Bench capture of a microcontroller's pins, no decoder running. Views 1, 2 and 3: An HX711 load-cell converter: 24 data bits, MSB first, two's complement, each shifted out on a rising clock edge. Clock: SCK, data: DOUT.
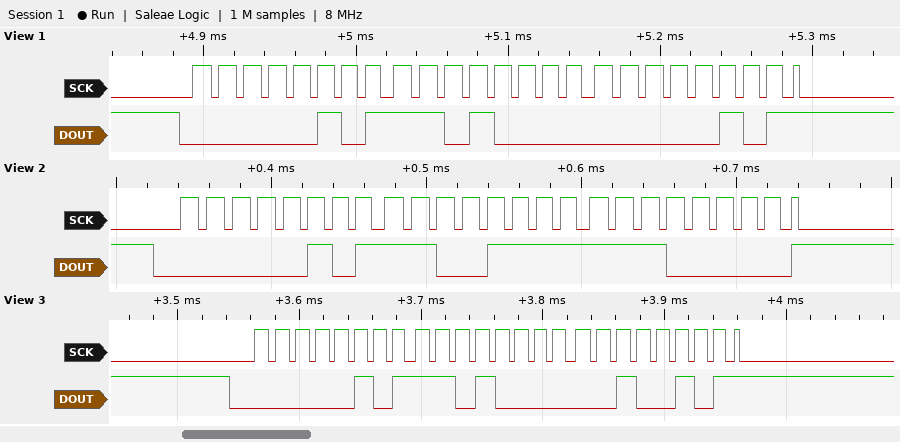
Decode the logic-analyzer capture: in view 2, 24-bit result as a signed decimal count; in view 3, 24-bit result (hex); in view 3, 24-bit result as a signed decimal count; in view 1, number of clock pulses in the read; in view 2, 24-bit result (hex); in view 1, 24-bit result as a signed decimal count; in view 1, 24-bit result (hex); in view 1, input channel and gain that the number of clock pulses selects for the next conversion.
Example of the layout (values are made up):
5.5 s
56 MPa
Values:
380896
0x05D025
380965
25
0x05CFE0
380933
0x05D005
channel A, gain 128
